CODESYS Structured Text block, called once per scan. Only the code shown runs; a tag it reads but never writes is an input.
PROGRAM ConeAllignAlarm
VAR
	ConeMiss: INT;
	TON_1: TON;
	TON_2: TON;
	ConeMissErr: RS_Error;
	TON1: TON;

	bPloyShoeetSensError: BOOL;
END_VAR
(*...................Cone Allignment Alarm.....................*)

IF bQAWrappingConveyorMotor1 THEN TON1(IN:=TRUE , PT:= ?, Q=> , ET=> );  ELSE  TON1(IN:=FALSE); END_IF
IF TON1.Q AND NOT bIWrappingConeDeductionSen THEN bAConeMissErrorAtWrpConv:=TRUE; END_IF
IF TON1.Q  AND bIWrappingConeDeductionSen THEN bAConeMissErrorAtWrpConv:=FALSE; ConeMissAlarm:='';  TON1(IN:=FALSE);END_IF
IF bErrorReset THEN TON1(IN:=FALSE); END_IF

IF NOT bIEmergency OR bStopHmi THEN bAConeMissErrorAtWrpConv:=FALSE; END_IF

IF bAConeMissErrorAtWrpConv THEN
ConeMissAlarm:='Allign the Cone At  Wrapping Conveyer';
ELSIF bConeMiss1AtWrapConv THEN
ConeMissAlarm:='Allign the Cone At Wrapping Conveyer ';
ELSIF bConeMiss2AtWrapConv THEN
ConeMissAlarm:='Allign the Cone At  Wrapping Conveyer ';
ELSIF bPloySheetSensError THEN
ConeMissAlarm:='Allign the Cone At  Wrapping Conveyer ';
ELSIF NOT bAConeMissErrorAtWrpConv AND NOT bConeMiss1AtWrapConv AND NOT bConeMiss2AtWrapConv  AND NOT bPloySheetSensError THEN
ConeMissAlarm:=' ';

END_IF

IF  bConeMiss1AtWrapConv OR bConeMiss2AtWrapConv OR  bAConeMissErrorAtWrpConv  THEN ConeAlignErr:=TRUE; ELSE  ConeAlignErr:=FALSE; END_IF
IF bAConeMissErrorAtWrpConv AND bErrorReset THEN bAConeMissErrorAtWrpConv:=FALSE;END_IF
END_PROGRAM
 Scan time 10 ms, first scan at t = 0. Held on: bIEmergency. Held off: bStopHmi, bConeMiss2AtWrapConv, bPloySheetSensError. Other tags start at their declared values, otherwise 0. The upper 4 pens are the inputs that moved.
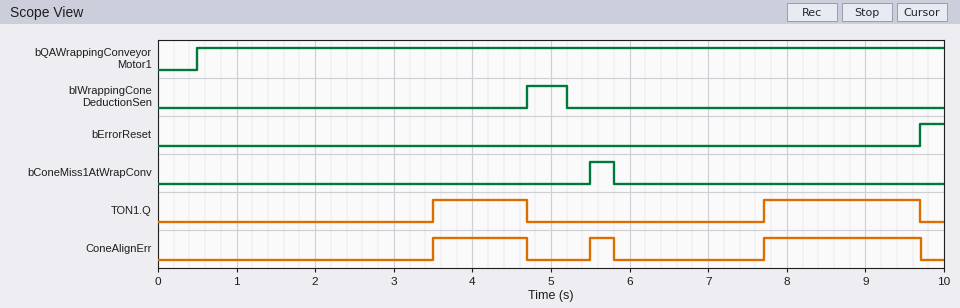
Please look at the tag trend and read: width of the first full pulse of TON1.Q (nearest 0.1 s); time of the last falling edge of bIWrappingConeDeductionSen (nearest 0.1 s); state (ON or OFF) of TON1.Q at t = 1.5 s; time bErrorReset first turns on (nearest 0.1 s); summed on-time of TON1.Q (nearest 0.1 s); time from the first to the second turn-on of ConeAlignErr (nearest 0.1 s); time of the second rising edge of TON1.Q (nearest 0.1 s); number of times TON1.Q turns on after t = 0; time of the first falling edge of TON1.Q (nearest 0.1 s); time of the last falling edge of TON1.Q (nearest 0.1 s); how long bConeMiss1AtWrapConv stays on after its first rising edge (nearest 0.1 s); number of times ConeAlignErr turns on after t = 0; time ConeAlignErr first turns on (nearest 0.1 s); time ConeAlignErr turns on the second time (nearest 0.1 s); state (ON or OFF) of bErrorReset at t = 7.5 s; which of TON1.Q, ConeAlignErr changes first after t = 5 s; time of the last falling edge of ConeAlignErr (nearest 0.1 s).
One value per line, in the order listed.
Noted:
1.2 s
5.2 s
OFF
9.7 s
3.2 s
2.0 s
7.7 s
2
4.7 s
9.7 s
0.3 s
3
3.5 s
5.5 s
OFF
ConeAlignErr
9.7 s
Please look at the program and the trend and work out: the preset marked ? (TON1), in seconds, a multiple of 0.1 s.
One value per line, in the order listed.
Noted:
3.0 s
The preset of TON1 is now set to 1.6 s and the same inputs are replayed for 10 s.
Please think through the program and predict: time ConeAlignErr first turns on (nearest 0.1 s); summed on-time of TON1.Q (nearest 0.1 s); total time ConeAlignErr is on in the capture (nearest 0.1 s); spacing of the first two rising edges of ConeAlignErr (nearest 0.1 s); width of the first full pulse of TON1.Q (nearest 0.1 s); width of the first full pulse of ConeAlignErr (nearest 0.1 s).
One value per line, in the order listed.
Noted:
2.1 s
6.0 s
6.3 s
3.4 s
2.6 s
2.6 s
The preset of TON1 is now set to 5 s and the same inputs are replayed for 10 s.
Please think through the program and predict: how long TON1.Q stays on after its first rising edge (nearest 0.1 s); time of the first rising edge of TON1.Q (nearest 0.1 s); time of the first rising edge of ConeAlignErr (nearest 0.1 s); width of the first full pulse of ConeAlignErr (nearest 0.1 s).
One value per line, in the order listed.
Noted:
4.2 s
5.5 s
5.5 s
4.2 s
